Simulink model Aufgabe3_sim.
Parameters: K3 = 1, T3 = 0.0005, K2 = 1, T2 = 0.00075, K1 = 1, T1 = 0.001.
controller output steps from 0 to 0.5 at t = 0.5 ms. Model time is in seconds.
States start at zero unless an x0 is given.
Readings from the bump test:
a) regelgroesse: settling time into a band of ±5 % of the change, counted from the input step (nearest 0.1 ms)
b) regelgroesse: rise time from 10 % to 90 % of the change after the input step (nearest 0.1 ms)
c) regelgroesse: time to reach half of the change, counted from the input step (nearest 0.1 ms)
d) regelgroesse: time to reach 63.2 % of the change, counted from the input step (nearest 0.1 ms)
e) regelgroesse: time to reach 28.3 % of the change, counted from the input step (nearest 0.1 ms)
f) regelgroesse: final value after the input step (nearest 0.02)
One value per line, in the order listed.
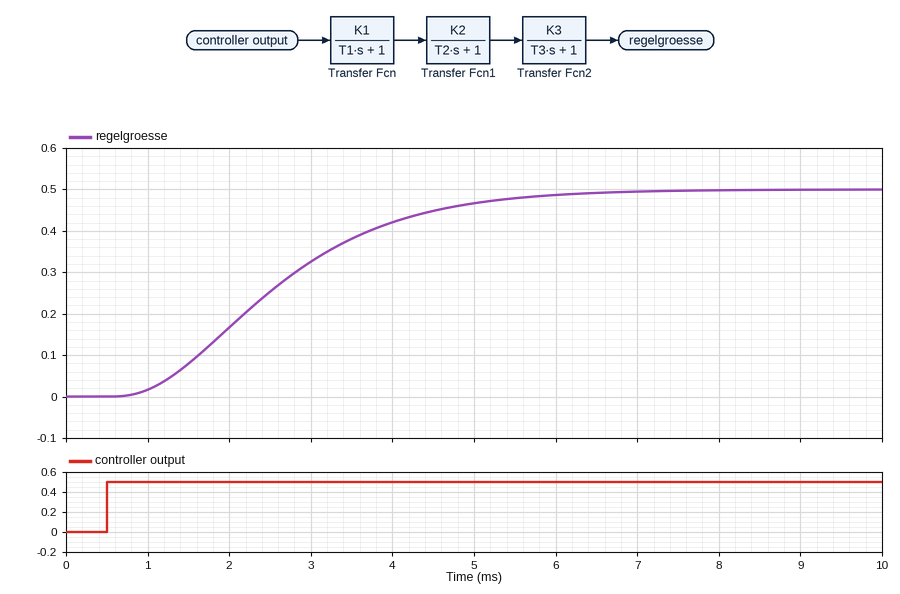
4.8 ms
3.2 ms
2.0 ms
2.4 ms
1.4 ms
0.50
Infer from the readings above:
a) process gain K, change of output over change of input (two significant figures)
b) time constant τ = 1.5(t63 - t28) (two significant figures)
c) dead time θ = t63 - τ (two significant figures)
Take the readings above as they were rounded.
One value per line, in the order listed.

1.0
1.5 ms
0.90 ms
